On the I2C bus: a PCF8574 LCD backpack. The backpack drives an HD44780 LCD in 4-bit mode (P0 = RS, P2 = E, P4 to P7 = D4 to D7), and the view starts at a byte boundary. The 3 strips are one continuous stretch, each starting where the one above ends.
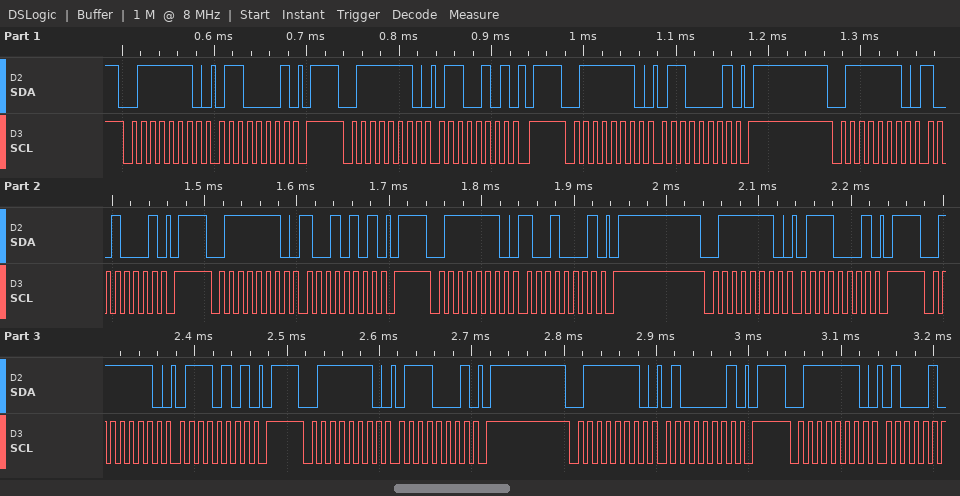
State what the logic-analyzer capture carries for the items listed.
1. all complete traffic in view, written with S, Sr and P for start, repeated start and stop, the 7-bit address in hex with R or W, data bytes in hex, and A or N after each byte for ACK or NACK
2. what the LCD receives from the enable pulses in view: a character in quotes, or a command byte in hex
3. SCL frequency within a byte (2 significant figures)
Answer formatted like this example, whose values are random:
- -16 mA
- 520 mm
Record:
- S 3FW A 61 A P S 3FW A 65 A P S 3FW A 61 A P S 3FW A 91 A P S 3FW A 95 A P S 3FW A 91 A P S 3FW A 71 A P S 3FW A 75 A P S 3FW A 71 A P S 3FW A 41 A P S 3FW A
- 'i'
- 100 kHz
